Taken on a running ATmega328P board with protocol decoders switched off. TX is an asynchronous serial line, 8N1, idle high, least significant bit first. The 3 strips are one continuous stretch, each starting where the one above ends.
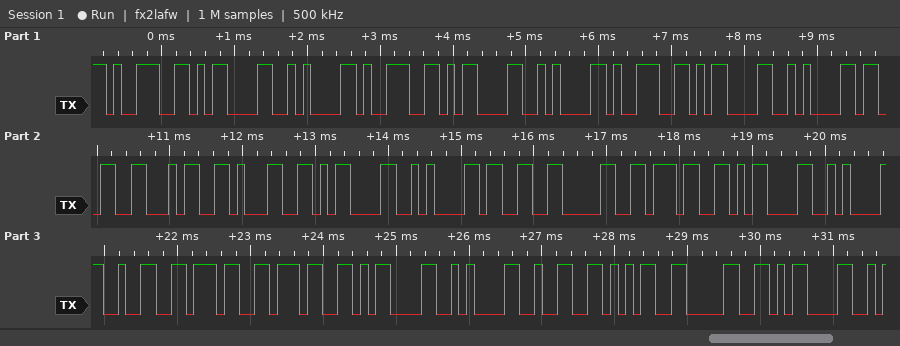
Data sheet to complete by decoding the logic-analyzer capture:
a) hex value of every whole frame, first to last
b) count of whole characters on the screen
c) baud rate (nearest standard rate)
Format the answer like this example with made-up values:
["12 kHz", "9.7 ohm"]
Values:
["0x39 0x0D 0x0A 0x39 0x0D 0x0A 0x39 0x0D 0x0A 0x33 0x34 0x31 0x0D 0x0A 0x33 0x30 0x37 0x0D 0x0A 0x32 0x37 0x37 0x0D 0x0A 0x32 0x35 0x30 0x0D", "28", "9600 baud"]
